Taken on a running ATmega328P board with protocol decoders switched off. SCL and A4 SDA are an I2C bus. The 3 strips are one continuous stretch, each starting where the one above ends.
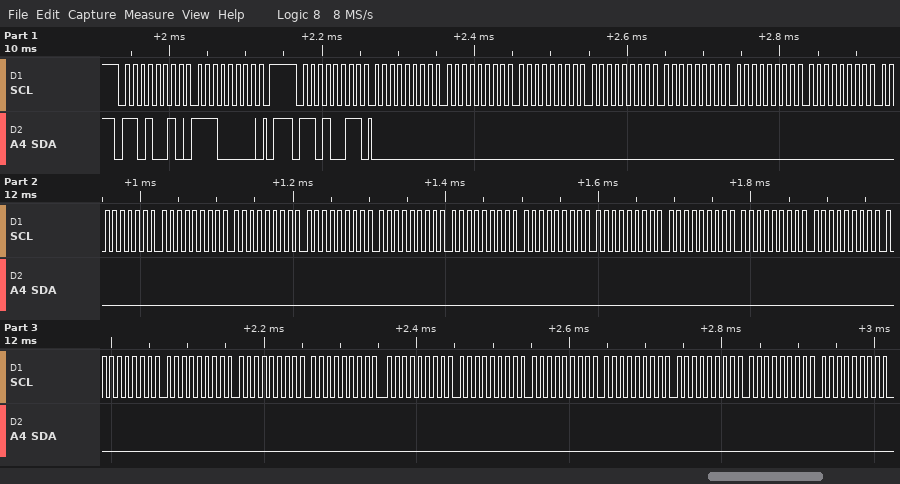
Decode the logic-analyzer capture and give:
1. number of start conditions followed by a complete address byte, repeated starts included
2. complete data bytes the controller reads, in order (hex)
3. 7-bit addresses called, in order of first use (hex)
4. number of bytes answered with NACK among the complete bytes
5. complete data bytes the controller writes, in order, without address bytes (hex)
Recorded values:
2
00 00 00 00 00 00 00 00 00 00 00 00 00 00 00 00 00 00 00 00 00 00 00 00 00 00 00 00 00
0x69
0
E0
